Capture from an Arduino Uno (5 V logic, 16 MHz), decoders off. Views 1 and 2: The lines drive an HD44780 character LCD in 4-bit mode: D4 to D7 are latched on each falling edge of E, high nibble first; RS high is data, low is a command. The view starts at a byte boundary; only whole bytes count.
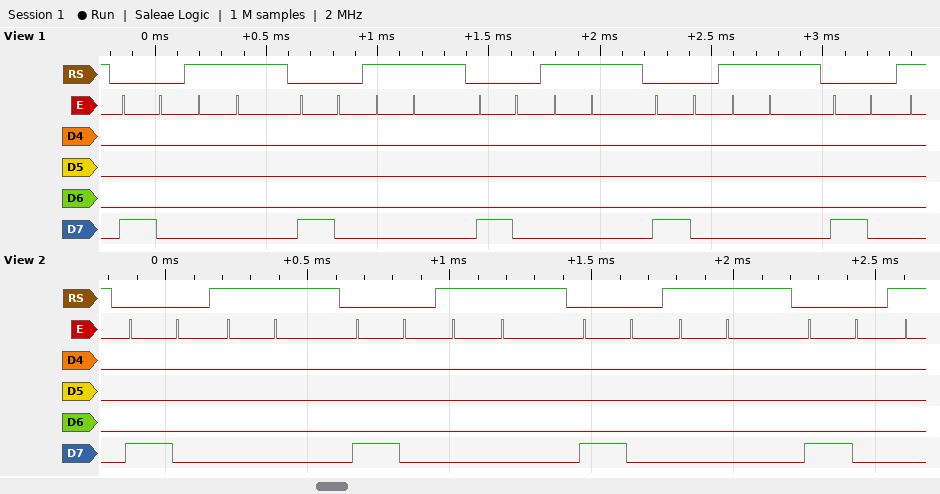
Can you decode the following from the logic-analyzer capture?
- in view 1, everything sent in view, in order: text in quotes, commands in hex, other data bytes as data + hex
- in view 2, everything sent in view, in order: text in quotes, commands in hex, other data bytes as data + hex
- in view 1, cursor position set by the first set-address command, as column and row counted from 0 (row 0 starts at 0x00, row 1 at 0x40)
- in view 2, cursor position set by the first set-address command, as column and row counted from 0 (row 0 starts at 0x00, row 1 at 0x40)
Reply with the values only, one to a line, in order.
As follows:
0x80 data 00 0x80 data 00 0x80 data 00 0x80 data 00 0x80
0x80 data 00 0x80 data 00 0x80 data 00 0x80
column 0, row 0
column 0, row 0
